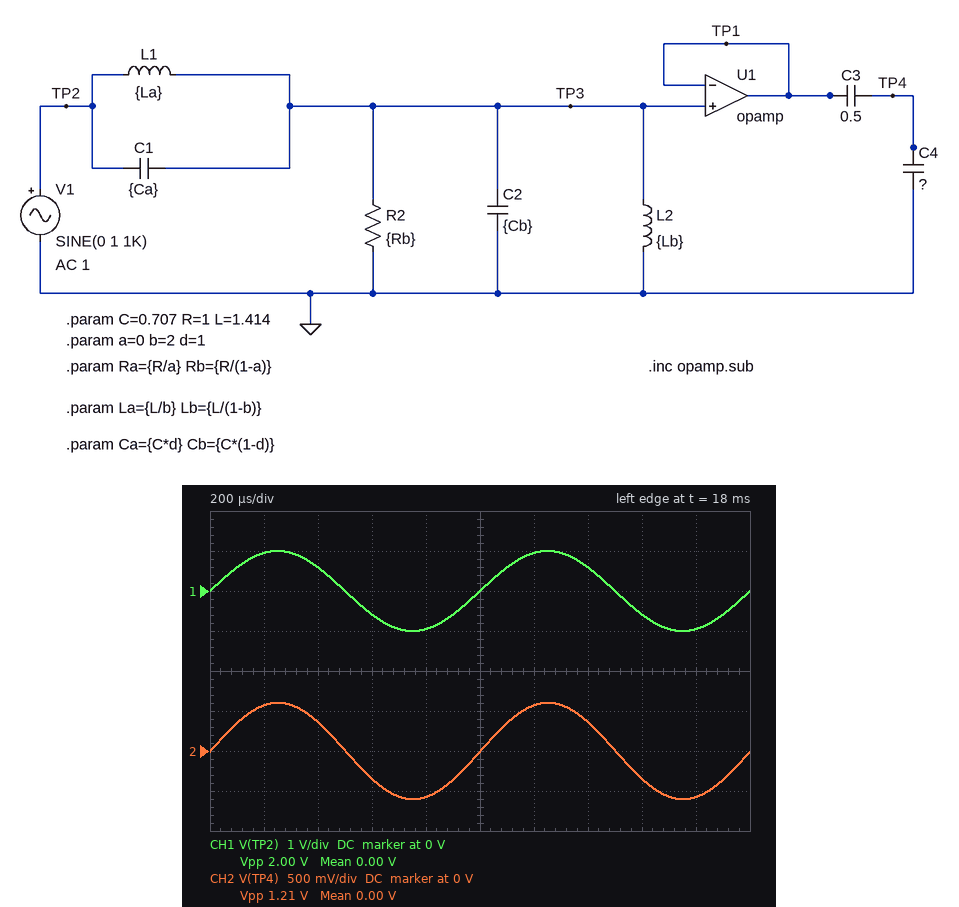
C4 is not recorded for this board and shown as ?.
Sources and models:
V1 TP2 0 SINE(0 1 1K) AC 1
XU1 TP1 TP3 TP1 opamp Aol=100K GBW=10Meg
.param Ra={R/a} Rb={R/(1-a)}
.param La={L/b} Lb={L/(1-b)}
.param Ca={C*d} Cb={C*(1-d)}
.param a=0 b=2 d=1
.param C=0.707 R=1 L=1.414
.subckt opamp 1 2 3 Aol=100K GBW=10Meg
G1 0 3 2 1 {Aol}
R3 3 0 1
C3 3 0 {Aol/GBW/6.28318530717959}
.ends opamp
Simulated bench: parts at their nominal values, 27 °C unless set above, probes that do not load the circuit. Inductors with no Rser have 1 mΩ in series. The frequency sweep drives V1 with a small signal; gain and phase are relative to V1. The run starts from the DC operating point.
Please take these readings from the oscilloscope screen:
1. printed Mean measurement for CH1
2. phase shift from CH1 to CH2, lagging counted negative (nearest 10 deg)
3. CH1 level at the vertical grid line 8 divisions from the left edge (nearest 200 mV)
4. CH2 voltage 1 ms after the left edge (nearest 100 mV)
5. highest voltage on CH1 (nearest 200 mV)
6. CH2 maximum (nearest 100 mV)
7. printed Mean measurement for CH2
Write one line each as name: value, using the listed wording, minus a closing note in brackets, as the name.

printed Mean measurement for CH1: 0.00 V
phase shift from CH1 to CH2, lagging counted negative: 0 deg
CH1 level at the vertical grid line 8 divisions from the left edge: -600 mV
CH2 voltage 1 ms after the left edge: 0 V
highest voltage on CH1: 1.0 V
CH2 maximum: 600 mV
printed Mean measurement for CH2: 0.00 V
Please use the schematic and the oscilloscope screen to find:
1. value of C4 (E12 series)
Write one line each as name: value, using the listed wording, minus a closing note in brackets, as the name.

value of C4: 330 mF
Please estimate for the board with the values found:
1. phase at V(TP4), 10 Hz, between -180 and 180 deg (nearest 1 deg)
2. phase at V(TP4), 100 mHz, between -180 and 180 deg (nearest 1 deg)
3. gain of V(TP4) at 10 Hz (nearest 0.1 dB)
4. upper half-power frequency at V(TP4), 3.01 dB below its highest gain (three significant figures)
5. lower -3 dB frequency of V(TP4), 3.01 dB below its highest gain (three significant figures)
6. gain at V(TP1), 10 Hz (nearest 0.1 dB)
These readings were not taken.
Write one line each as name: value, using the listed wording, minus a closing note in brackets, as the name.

phase at V(TP4), 10 Hz, between -180 and 180 deg: 1 deg
phase at V(TP4), 100 mHz, between -180 and 180 deg: -56 deg
gain of V(TP4) at 10 Hz: -4.4 dB
upper half-power frequency at V(TP4), 3.01 dB below its highest gain: 107 mHz
lower -3 dB frequency of V(TP4), 3.01 dB below its highest gain: 417 µHz
gain at V(TP1), 10 Hz: 0 dB
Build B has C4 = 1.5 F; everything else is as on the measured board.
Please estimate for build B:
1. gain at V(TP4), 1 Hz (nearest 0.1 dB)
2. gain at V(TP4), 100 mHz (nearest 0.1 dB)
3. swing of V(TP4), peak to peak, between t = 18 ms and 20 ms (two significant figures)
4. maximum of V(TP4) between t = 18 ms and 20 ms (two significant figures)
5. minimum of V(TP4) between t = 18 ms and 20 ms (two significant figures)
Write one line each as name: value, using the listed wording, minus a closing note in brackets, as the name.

gain at V(TP4), 1 Hz: -12.5 dB
gain at V(TP4), 100 mHz: -8.6 dB
swing of V(TP4), peak to peak, between t = 18 ms and 20 ms: 500 mV
maximum of V(TP4) between t = 18 ms and 20 ms: 250 mV
minimum of V(TP4) between t = 18 ms and 20 ms: -250 mV
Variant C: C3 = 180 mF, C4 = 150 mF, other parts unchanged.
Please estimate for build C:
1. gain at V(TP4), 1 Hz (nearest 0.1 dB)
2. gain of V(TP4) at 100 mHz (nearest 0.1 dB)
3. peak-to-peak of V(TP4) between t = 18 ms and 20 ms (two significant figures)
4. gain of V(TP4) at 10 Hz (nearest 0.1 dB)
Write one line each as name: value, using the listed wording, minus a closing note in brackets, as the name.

gain at V(TP4), 1 Hz: -5.7 dB
gain of V(TP4) at 100 mHz: -1.8 dB
peak-to-peak of V(TP4) between t = 18 ms and 20 ms: 1.1 V
gain of V(TP4) at 10 Hz: -5.3 dB
